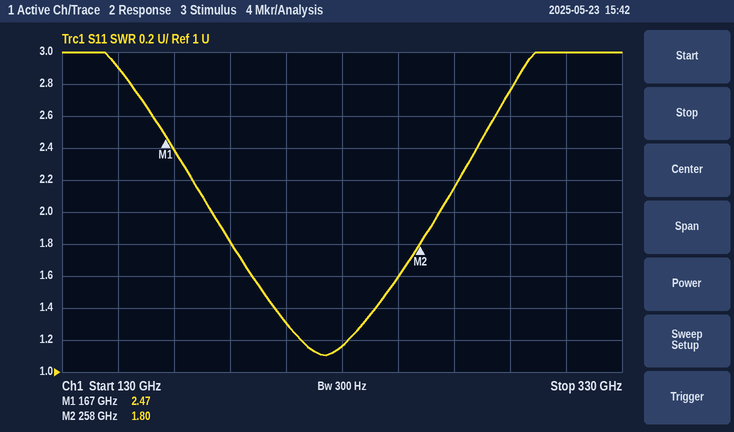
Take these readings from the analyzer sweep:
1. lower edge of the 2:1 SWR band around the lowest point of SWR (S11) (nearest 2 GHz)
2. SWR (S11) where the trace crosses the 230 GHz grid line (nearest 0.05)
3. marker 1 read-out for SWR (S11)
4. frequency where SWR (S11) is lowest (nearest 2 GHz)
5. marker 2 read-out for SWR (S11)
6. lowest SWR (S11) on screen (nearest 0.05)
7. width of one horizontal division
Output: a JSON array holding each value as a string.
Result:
["184 GHz", "1.15", "2.47", "224 GHz", "1.80", "1.10", "20 GHz"]
